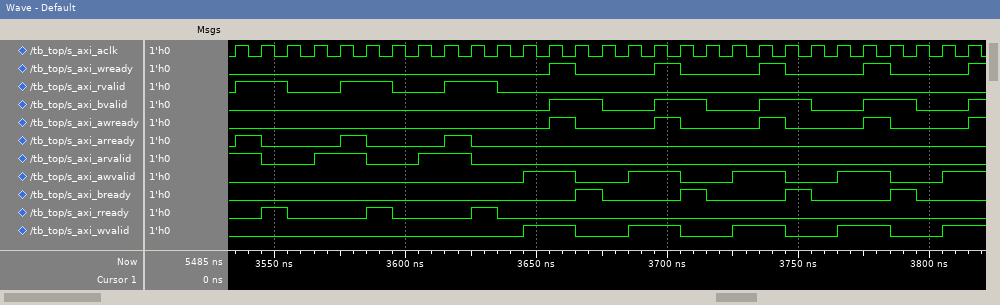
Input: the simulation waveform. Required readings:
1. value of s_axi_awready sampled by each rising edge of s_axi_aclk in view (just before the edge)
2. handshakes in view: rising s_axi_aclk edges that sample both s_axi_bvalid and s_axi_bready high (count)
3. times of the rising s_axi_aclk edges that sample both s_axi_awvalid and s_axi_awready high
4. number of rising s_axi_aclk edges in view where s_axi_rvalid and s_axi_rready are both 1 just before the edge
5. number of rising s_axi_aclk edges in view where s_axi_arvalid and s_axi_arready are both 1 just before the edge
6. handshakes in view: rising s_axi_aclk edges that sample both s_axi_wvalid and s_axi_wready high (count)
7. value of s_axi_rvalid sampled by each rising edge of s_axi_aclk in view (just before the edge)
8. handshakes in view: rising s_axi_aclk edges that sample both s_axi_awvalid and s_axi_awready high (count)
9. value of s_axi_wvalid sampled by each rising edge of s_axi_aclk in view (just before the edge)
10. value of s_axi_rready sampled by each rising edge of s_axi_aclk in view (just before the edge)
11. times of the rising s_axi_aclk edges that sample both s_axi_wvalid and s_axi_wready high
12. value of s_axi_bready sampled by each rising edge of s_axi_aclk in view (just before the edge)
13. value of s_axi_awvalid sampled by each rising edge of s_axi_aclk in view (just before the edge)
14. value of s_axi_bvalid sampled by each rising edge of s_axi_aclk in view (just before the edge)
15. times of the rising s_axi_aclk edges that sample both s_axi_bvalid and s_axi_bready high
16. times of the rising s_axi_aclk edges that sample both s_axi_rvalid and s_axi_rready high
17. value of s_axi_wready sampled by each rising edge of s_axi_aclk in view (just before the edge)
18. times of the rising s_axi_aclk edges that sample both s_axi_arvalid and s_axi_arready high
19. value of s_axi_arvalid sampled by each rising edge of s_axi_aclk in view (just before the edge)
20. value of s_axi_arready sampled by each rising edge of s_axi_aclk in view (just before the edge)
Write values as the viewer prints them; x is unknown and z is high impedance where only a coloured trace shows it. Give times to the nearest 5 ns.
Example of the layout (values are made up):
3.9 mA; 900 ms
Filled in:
0 0 0 0 0 0 0 0 0 0 0 0 0 1 0 0 0 1 0 0 0 1 0 0 0 1 0 0 0; 4; 3665 ns, 3705 ns, 3745 ns, 3785 ns; 3; 3; 4; 0 1 1 0 0 1 1 0 0 1 1 0 0 0 0 0 0 0 0 0 0 0 0 0 0 0 0 0 0; 4; 0 0 0 0 0 0 0 0 0 0 0 0 1 1 0 0 1 1 0 0 1 1 0 0 1 1 0 0 1; 0 0 1 0 0 0 1 0 0 0 1 0 0 0 0 0 0 0 0 0 0 0 0 0 0 0 0 0 0; 3665 ns, 3705 ns, 3745 ns, 3785 ns; 0 0 0 0 0 0 0 0 0 0 0 0 0 0 1 0 0 0 1 0 0 0 1 0 0 0 1 0 0; 0 0 0 0 0 0 0 0 0 0 0 0 1 1 0 0 1 1 0 0 1 1 0 0 1 1 0 0 1; 0 0 0 0 0 0 0 0 0 0 0 0 0 1 1 0 0 1 1 0 0 1 1 0 0 1 1 0 0; 3675 ns, 3715 ns, 3755 ns, 3795 ns; 3555 ns, 3595 ns, 3635 ns; 0 0 0 0 0 0 0 0 0 0 0 0 0 1 0 0 0 1 0 0 0 1 0 0 0 1 0 0 0; 3545 ns, 3585 ns, 3625 ns; 1 1 0 0 1 1 0 0 1 1 0 0 0 0 0 0 0 0 0 0 0 0 0 0 0 0 0 0 0; 0 1 0 0 0 1 0 0 0 1 0 0 0 0 0 0 0 0 0 0 0 0 0 0 0 0 0 0 0
